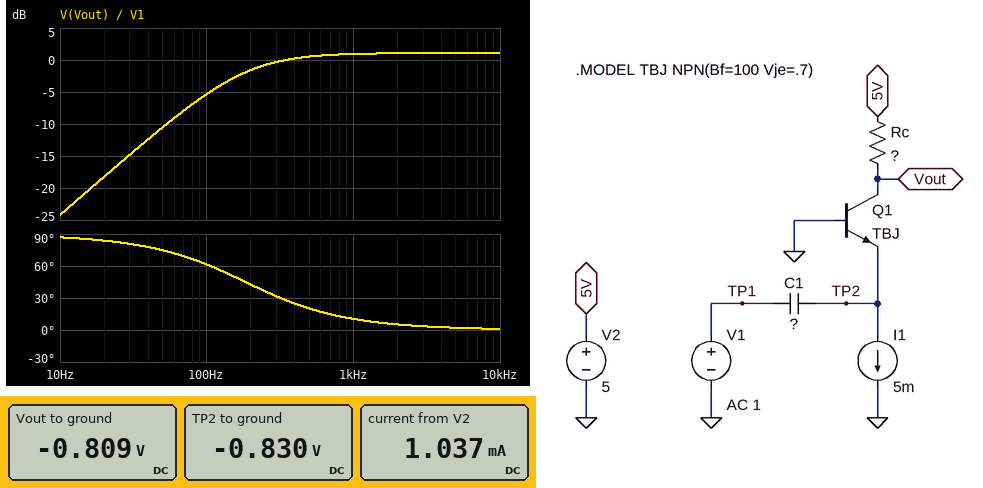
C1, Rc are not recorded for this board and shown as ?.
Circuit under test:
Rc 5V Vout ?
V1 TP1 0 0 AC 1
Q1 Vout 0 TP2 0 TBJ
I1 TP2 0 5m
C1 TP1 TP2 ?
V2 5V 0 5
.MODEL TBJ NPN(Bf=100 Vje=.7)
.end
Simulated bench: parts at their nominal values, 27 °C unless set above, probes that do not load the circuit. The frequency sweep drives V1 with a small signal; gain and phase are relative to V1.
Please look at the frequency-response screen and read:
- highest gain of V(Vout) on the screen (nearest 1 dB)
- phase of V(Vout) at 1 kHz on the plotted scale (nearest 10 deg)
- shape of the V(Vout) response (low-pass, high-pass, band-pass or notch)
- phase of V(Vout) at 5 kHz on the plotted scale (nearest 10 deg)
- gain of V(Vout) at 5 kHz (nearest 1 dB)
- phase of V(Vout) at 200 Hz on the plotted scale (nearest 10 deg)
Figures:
1 dB
10 deg
high-pass
0 deg
1 dB
40 deg
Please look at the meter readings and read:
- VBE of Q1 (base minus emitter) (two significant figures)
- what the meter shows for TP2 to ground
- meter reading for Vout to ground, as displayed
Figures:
830 mV
-0.830 V
-0.809 V
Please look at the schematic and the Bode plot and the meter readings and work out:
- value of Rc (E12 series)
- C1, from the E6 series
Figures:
5.6 kΩ
150 µF
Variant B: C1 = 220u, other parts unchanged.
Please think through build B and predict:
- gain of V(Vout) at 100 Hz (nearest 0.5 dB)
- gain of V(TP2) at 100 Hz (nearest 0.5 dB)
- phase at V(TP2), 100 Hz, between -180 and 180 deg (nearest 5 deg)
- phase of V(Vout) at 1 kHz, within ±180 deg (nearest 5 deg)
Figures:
-3.0 dB
-4.0 dB
50 deg
5 deg
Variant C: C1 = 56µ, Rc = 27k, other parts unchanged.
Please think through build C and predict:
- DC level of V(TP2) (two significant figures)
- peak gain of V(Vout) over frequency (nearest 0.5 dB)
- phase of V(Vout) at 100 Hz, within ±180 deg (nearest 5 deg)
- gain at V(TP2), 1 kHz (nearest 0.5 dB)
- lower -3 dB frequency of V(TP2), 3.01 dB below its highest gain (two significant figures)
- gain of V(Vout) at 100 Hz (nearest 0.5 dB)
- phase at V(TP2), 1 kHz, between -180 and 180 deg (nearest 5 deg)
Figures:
-830 mV
0 dB
80 deg
-1.0 dB
540 Hz
-14.5 dB
30 deg
